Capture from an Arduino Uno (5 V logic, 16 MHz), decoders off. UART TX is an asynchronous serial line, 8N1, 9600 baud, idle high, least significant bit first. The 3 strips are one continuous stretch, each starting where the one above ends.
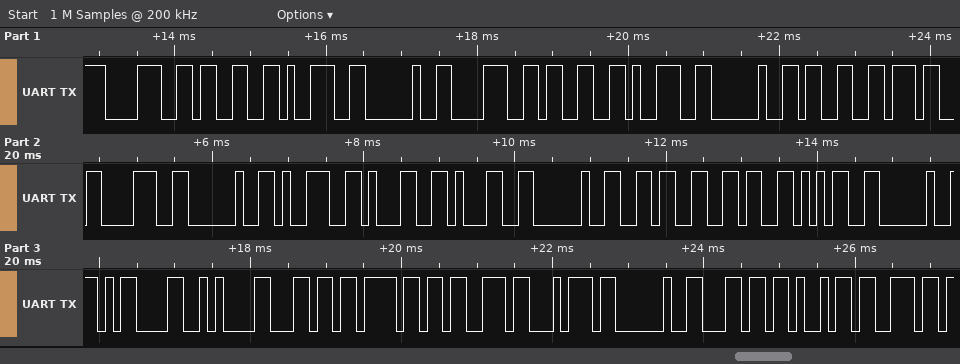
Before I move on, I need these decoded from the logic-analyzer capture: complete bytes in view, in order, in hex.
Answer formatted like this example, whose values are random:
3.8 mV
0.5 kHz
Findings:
0x38 0x33 0x39 0x20 0x38 0x33 0x39 0x20 0x33 0x37 0x38 0x20 0x39 0x31 0x31 0x20 0x36 0x36 0x35 0x20 0x0D 0x0A 0x6C 0x6F 0x73 0x74 0x20 0x6C 0x69 0x6E
